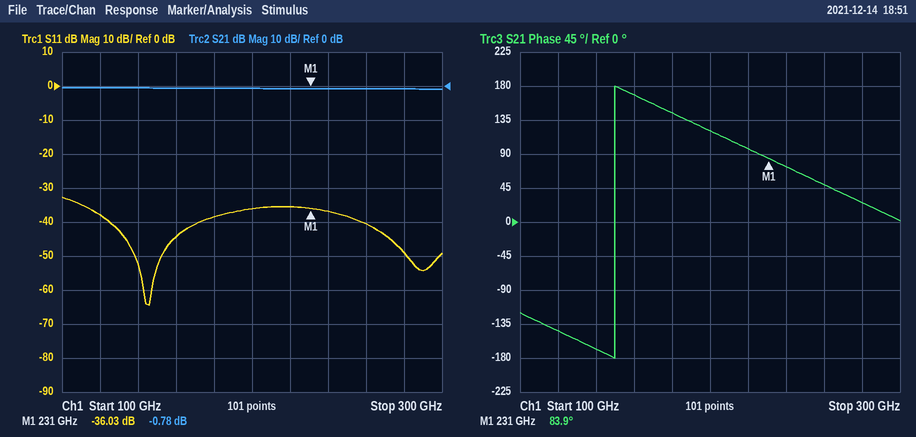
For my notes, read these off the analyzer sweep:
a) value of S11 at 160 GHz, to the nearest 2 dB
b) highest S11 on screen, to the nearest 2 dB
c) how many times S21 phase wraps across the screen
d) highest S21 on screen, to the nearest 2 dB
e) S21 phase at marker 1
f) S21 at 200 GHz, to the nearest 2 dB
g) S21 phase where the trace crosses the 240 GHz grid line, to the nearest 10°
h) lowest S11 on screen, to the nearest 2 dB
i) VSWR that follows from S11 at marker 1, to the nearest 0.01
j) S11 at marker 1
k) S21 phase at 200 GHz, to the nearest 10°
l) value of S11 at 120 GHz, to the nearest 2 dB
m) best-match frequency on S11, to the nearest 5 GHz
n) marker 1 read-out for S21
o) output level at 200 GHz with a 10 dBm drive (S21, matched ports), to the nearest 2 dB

-44 dB
-32 dB
1
0 dB
83.9°
0 dB
70°
-64 dB
1.03
-36.03 dB
120°
-38 dB
145 GHz
-0.78 dB
10 dBm
